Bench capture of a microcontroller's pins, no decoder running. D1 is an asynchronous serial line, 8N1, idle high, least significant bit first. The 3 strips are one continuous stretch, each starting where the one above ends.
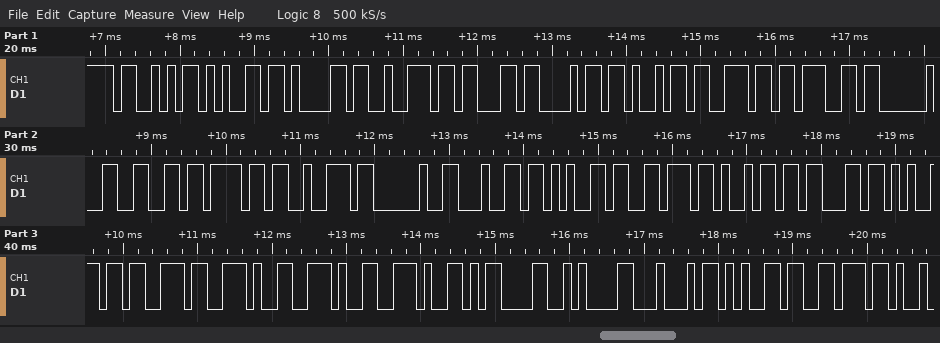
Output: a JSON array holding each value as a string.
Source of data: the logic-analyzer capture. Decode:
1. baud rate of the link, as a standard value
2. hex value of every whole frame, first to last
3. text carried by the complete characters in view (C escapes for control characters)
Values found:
["9600 baud", "0x53 0x65 0x61 0x72 0x63 0x68 0x69 0x6E 0x67 0x20 0x66 0x6F 0x72 0x20 0x64 0x65 0x76 0x69 0x63 0x65 0x73 0x2E 0x2E 0x2E 0x0D 0x0A 0x44 0x65 0x76", "\"Searching for devices...\\r\\nDev\""]
